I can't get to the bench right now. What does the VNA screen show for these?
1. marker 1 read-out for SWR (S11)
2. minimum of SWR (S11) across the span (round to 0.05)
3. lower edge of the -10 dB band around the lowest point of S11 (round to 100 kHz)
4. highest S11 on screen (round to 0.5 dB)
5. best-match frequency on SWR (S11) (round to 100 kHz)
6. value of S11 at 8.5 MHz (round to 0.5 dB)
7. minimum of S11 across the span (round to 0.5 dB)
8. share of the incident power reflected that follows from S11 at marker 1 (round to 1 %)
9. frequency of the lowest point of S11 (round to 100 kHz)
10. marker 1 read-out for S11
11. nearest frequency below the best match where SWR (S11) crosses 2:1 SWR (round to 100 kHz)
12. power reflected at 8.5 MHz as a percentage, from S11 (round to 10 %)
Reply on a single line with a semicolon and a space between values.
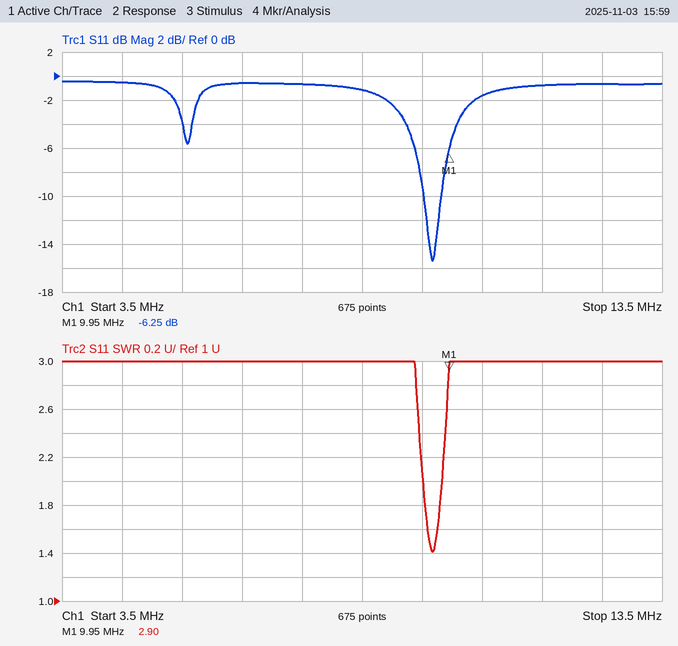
2.90; 1.40; 9.5 MHz; -0.5 dB; 9.7 MHz; -1.0 dB; -15.5 dB; 24 %; 9.7 MHz; -6.25 dB; 9.5 MHz; 80 %
